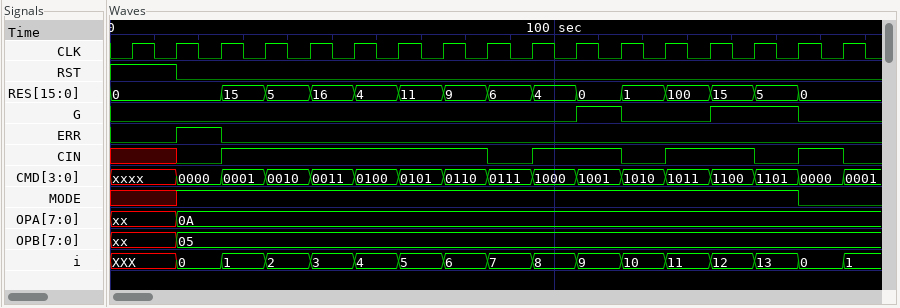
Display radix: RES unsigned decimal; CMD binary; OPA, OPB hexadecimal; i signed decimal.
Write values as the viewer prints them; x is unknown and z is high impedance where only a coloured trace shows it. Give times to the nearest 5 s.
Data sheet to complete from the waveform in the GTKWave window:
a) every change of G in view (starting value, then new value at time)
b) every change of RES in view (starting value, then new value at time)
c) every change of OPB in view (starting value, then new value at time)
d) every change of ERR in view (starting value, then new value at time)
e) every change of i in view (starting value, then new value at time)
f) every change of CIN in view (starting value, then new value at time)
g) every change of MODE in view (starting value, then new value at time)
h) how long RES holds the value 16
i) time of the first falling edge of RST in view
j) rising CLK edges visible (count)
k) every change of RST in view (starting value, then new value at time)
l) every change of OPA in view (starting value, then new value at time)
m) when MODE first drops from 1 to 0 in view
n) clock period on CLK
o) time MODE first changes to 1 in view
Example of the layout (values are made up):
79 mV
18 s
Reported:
0, 1 at 105 s, 0 at 115 s, 1 at 135 s, 0 at 155 s
0, 15 at 25 s, 5 at 35 s, 16 at 45 s, 4 at 55 s, 11 at 65 s, 9 at 75 s, 6 at 85 s, 4 at 95 s, 0 at 105 s, 1 at 115 s, 100 at 125 s, 15 at 135 s, 5 at 145 s, 0 at 155 s
xx, 05 at 15 s
0, 1 at 15 s, 0 at 25 s
XXX, 0 at 15 s, 1 at 25 s, 2 at 35 s, 3 at 45 s, 4 at 55 s, 5 at 65 s, 6 at 75 s, 7 at 85 s, 8 at 95 s, 9 at 105 s, 10 at 115 s, 11 at 125 s, 12 at 135 s, 13 at 145 s, 0 at 155 s, 1 at 165 s
x, 0 at 15 s, 1 at 25 s, 0 at 85 s, 1 at 95 s, 0 at 115 s, 1 at 125 s, 0 at 145 s, 1 at 155 s, 0 at 165 s
x, 1 at 15 s, 0 at 155 s
10 s
15 s
17
1, 0 at 15 s
xx, 0A at 15 s
155 s
10 s
15 s
